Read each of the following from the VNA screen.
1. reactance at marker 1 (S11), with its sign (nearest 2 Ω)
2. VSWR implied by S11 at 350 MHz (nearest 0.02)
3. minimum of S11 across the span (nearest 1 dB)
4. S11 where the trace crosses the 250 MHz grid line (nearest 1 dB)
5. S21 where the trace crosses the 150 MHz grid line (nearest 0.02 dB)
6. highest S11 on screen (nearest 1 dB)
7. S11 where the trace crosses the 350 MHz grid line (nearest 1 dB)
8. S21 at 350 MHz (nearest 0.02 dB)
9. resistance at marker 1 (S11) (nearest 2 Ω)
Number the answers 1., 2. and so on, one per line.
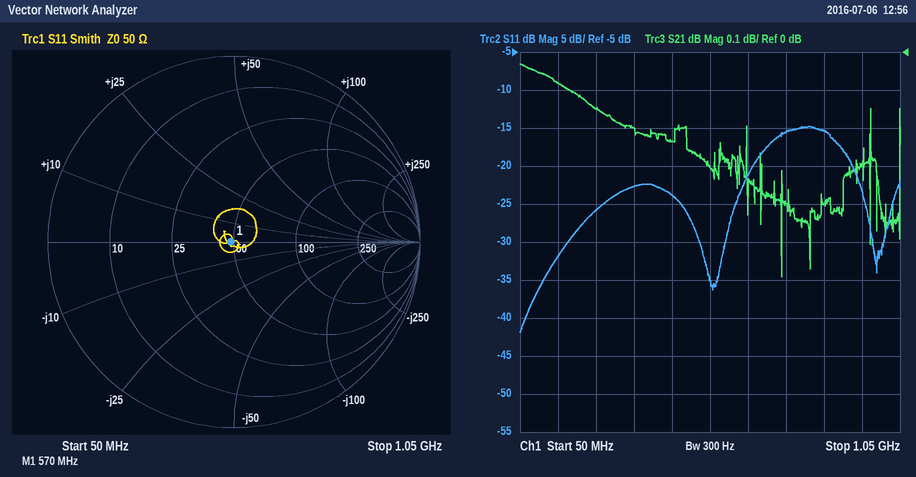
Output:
1. 0 Ω
2. 1.16
3. -42 dB
4. -26 dB
5. -0.08 dB
6. -15 dB
7. -23 dB
8. -0.20 dB
9. 48 Ω
